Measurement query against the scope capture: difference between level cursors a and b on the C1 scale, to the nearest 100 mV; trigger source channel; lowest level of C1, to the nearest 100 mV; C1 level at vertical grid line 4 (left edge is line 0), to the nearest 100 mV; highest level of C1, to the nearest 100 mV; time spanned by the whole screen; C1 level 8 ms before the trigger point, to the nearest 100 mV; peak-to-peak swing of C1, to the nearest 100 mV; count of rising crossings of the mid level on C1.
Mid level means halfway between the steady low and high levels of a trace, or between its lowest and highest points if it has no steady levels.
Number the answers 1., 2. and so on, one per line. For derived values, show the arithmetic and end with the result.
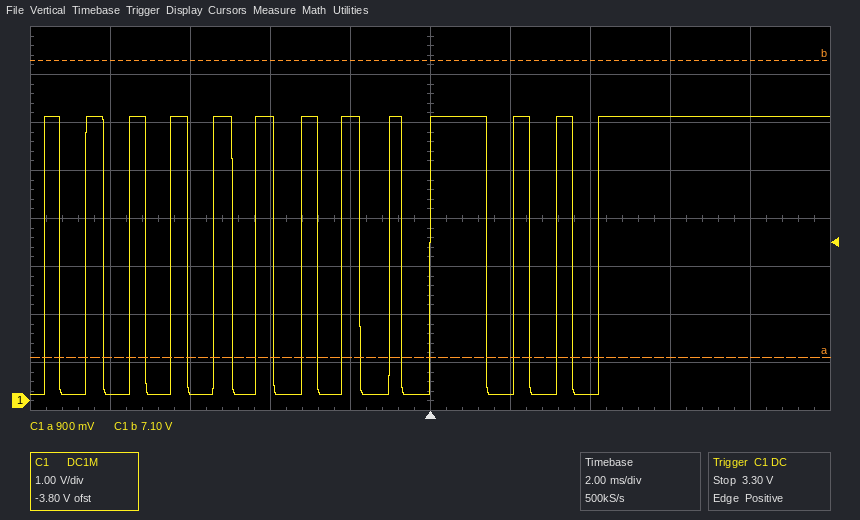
1. 6.2 V
2. C1
3. 100 mV
4. 5.9 V
5. 5.9 V
6. 20 ms
7. 100 mV
8. 5.9 V − (100 mV) = 5.8 V
9. 13
